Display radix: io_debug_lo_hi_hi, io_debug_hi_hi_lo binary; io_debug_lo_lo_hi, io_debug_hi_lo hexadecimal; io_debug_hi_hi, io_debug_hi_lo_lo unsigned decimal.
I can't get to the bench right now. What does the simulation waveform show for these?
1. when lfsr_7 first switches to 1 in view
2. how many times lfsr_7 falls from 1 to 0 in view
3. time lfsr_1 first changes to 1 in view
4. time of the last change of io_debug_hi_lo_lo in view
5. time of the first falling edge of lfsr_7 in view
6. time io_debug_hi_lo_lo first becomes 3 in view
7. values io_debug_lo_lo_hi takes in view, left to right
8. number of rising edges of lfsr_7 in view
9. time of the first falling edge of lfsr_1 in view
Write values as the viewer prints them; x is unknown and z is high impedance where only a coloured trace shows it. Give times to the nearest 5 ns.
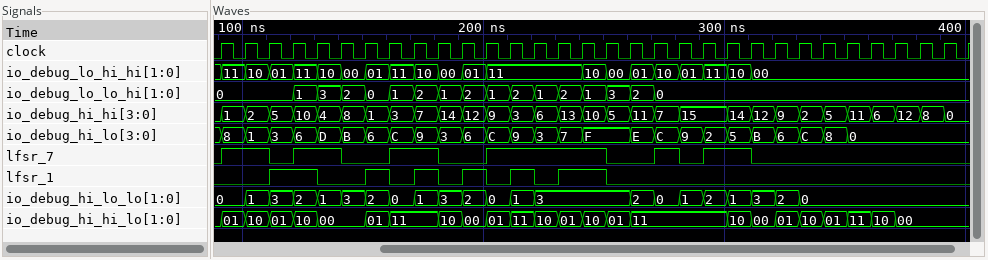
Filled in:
90 ns
6
110 ns
330 ns
110 ns
110 ns
0, 1, 3, 2, 0, 1, 2, 1, 2, 1, 2, 1, 2, 1, 3, 2, 0
6
130 ns
